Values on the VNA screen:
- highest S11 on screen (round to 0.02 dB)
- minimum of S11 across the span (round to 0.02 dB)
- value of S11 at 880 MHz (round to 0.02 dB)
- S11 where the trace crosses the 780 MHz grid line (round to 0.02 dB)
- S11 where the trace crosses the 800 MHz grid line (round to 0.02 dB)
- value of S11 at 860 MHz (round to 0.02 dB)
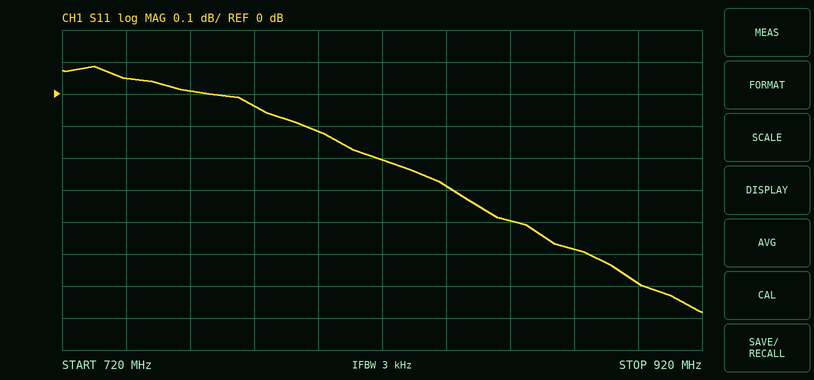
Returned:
0.08 dB
-0.68 dB
-0.48 dB
-0.04 dB
-0.12 dB
-0.40 dB
